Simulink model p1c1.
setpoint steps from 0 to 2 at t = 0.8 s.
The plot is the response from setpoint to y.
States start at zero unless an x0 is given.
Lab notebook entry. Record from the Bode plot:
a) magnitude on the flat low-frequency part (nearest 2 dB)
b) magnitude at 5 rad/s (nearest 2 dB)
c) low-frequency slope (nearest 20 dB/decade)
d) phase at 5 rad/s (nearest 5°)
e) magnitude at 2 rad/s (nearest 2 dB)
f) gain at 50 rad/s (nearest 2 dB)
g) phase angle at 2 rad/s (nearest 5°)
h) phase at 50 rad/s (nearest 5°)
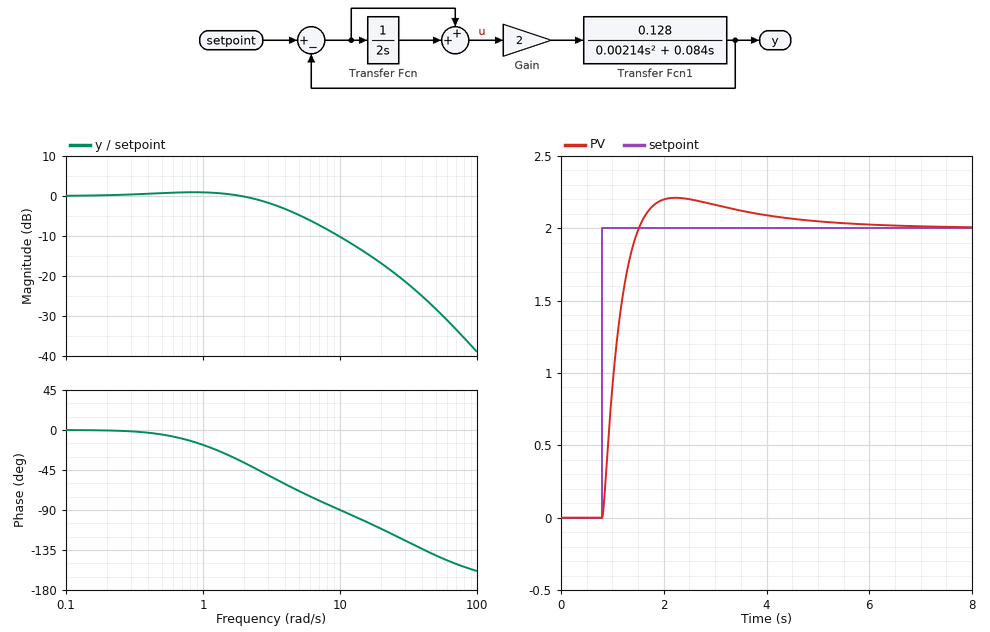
0 dB
-4 dB
0 dB/decade
-70°
0 dB
-28 dB
-35°
-140°
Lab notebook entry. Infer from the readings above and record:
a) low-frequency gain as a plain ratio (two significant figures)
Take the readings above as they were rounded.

1.0
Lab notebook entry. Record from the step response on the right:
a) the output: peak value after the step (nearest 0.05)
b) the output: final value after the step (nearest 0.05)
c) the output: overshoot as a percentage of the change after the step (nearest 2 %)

2.20
2.00
10 %
